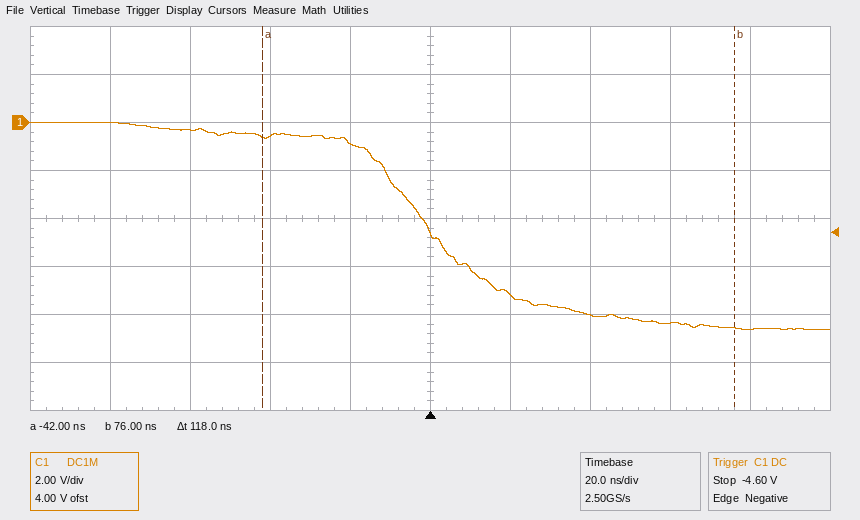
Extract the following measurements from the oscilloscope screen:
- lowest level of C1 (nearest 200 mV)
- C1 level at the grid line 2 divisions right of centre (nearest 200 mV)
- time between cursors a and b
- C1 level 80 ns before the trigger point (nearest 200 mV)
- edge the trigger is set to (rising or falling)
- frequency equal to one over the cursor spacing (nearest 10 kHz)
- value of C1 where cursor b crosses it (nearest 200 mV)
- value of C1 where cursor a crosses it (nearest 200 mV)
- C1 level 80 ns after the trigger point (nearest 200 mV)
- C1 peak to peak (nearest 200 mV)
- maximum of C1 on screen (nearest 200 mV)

-8.6 V
-8.0 V
118 ns
0.0 V
falling
8.47 MHz
-8.6 V
-600 mV
-8.6 V
8.6 V
0.0 V
